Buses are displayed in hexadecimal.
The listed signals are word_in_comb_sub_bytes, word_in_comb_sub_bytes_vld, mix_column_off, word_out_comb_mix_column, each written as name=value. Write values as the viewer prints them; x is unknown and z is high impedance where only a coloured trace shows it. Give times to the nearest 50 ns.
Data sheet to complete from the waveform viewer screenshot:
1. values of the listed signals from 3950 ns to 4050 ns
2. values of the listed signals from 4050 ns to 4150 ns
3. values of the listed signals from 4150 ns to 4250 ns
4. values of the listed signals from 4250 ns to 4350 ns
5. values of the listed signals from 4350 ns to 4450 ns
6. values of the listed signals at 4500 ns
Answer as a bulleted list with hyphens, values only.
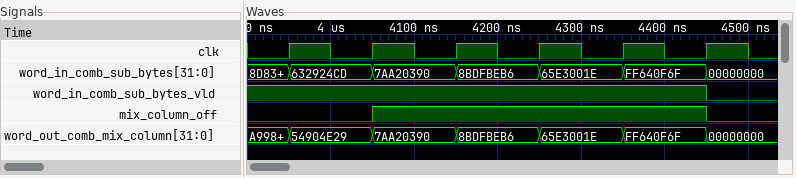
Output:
- word_in_comb_sub_bytes=632924CD, word_in_comb_sub_bytes_vld=1, mix_column_off=0, word_out_comb_mix_column=54904E29
- word_in_comb_sub_bytes=7AA20390, word_in_comb_sub_bytes_vld=1, mix_column_off=1, word_out_comb_mix_column=7AA20390
- word_in_comb_sub_bytes=8BDFBEB6, word_in_comb_sub_bytes_vld=1, mix_column_off=1, word_out_comb_mix_column=8BDFBEB6
- word_in_comb_sub_bytes=65E3001E, word_in_comb_sub_bytes_vld=1, mix_column_off=1, word_out_comb_mix_column=65E3001E
- word_in_comb_sub_bytes=FF640F6F, word_in_comb_sub_bytes_vld=1, mix_column_off=1, word_out_comb_mix_column=FF640F6F
- word_in_comb_sub_bytes=00000000, word_in_comb_sub_bytes_vld=0, mix_column_off=0, word_out_comb_mix_column=00000000
